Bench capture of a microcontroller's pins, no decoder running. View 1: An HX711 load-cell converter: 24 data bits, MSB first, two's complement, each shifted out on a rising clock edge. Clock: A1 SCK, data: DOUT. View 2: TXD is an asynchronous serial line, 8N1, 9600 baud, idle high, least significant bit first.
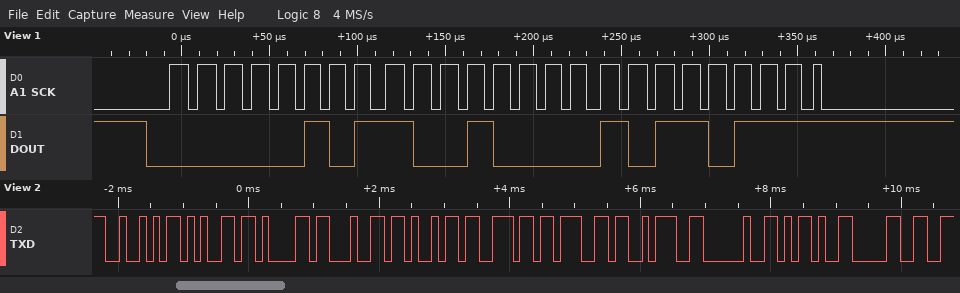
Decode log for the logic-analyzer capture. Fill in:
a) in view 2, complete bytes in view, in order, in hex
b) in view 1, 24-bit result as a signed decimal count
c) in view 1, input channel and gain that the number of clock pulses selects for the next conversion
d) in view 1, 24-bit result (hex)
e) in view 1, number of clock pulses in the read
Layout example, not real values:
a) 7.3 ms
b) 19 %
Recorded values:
a) 52 65 61 64 69 6E 67 3A 20 2D 30
b) 364727
c) channel A, gain 128
d) 0x0590B7
e) 25
